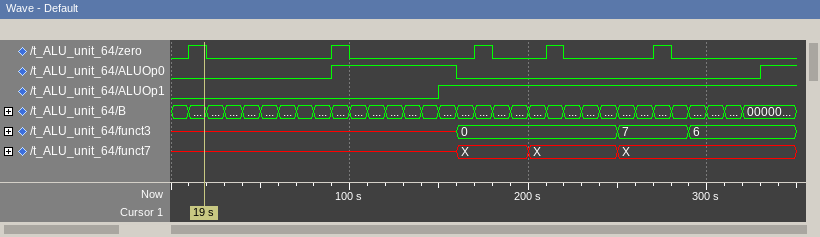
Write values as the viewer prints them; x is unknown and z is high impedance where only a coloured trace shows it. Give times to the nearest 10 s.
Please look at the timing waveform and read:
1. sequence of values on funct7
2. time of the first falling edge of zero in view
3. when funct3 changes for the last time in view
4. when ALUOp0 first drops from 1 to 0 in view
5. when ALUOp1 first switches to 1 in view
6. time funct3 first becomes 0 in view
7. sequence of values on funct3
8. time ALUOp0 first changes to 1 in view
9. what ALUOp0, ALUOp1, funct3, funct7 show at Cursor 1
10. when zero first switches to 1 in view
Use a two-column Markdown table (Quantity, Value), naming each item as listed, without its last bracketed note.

| Quantity | Value |
|---|---|
| sequence of values on funct7 | x, X, X, X |
| time of the first falling edge of zero in view | 20 s |
| when funct3 changes for the last time in view | 290 s |
| when ALUOp0 first drops from 1 to 0 in view | 160 s |
| when ALUOp1 first switches to 1 in view | 150 s |
| time funct3 first becomes 0 in view | 160 s |
| sequence of values on funct3 | x, 0, 7, 6 |
| time ALUOp0 first changes to 1 in view | 90 s |
| what ALUOp0, ALUOp1, funct3, funct7 show at Cursor 1 | ALUOp0=0, ALUOp1=0, funct3=x, funct7=x |
| when zero first switches to 1 in view | 10 s |
